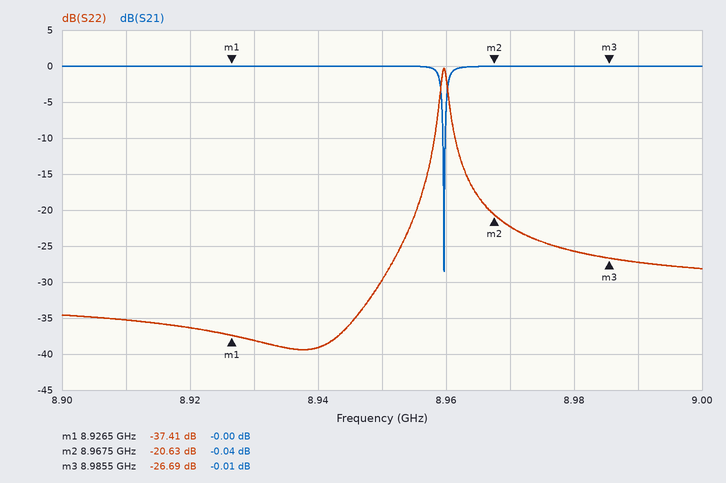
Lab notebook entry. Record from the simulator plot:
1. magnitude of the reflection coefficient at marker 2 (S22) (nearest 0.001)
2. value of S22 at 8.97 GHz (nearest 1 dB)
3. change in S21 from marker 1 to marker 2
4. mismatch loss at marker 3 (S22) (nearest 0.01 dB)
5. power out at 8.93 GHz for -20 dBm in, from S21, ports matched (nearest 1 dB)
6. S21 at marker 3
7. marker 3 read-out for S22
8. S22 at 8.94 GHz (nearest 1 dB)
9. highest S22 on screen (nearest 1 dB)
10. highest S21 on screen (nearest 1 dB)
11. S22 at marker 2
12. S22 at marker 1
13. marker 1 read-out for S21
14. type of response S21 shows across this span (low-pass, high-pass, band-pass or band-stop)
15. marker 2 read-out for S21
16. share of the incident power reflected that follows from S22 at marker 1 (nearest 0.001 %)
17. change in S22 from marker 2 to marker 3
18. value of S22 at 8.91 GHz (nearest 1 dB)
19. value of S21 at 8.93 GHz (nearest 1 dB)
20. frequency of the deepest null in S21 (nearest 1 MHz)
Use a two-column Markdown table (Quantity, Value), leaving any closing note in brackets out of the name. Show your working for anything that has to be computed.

| Quantity | Value |
|---|---|
| magnitude of the reflection coefficient at marker 2 (S22) | 10^(-20.63/20) ≈ 0.093 |
| value of S22 at 8.97 GHz | -22 dB |
| change in S21 from marker 1 to marker 2 | -0.04 − (-0) = -0.04 dB |
| mismatch loss at marker 3 (S22) | −10 log10(1 − 10^(-26.69/10)) ≈ 0.01 dB |
| power out at 8.93 GHz for -20 dBm in, from S21, ports matched | -20 dBm + (0 dB) = -20 dBm |
| S21 at marker 3 | -0.01 dB |
| marker 3 read-out for S22 | -26.69 dB |
| S22 at 8.94 GHz | -39 dB |
| highest S22 on screen | 0 dB |
| highest S21 on screen | 0 dB |
| S22 at marker 2 | -20.63 dB |
| S22 at marker 1 | -37.41 dB |
| marker 1 read-out for S21 | -0.00 dB |
| type of response S21 shows across this span | band-stop |
| marker 2 read-out for S21 | -0.04 dB |
| share of the incident power reflected that follows from S22 at marker 1 | 10^(-37.41/10) ≈ 0.018 % |
| change in S22 from marker 2 to marker 3 | -26.69 − (-20.63) = -6.06 dB |
| value of S22 at 8.91 GHz | -35 dB |
| value of S21 at 8.93 GHz | 0 dB |
| frequency of the deepest null in S21 | 8.960 GHz |
